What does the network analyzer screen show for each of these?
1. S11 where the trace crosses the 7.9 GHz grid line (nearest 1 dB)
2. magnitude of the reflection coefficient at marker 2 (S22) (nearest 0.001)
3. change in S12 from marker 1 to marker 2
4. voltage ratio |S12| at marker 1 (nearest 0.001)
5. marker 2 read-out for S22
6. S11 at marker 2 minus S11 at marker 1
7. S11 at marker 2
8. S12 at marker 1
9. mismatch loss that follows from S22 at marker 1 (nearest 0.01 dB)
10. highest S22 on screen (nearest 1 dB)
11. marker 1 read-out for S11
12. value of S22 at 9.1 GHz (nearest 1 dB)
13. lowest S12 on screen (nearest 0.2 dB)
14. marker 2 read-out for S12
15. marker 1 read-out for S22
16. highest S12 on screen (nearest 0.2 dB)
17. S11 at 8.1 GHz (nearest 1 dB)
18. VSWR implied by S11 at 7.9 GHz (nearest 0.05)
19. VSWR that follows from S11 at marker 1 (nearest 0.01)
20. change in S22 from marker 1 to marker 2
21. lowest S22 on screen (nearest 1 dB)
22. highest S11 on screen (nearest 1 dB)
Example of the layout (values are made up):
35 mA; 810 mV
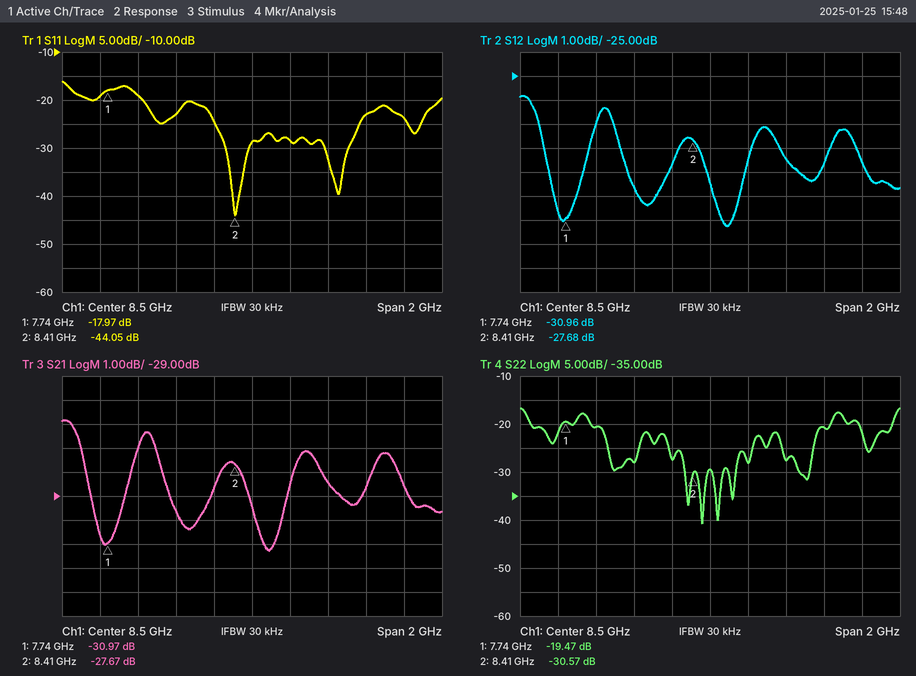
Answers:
-19 dB; 0.030; 3.28 dB; 0.028; -30.57 dB; -26.08 dB; -44.05 dB; -30.96 dB; 0.05 dB; -17 dB; -17.97 dB; -21 dB; -31.2 dB; -27.68 dB; -19.47 dB; -25.8 dB; -23 dB; 1.25; 1.29; -11.10 dB; -41 dB; -16 dB
